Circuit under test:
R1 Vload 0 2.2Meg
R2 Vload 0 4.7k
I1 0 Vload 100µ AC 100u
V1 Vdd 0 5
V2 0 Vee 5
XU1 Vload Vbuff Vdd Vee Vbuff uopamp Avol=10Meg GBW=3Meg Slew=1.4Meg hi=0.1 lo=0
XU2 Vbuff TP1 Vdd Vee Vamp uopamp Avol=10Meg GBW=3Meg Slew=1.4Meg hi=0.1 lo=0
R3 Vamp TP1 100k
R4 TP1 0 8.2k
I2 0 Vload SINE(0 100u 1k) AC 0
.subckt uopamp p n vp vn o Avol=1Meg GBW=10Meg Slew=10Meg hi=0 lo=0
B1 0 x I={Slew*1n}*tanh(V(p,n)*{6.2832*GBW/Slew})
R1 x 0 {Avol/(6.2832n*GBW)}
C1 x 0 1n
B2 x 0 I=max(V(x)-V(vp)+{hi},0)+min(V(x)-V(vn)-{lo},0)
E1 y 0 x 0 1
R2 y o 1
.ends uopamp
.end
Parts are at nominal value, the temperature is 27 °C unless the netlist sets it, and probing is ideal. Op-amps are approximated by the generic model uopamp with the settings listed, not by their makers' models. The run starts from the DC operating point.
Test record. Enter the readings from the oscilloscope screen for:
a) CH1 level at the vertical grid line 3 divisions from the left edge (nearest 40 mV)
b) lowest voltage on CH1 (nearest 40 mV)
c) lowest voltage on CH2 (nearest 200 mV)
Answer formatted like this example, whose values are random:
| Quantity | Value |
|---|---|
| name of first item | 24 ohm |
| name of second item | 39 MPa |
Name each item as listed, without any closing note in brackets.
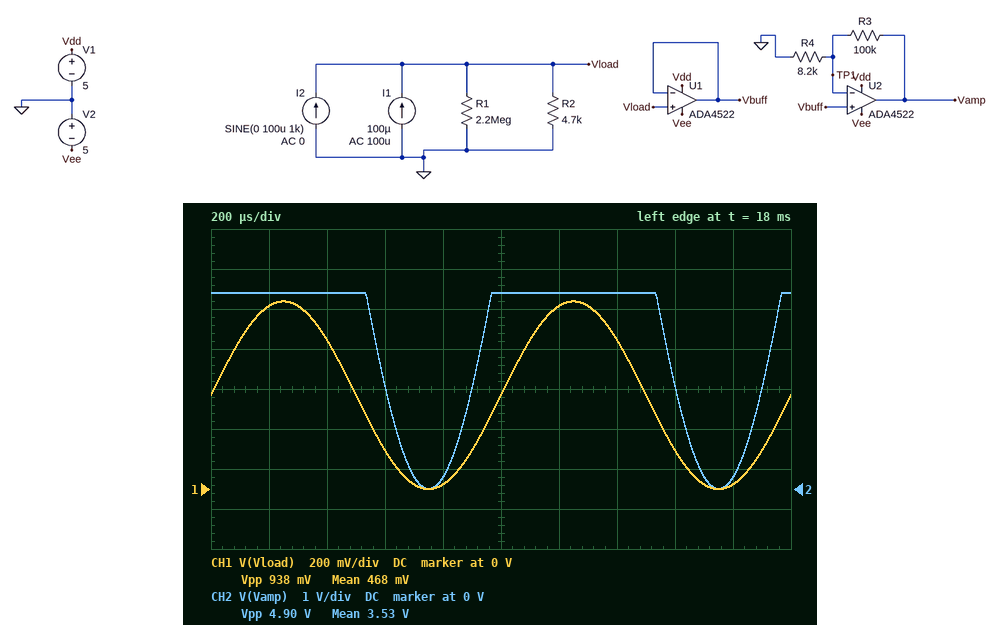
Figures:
| Quantity | Value |
|---|---|
| CH1 level at the vertical grid line 3 divisions from the left edge | 200 mV |
| lowest voltage on CH1 | 0 V |
| lowest voltage on CH2 | 0 V |
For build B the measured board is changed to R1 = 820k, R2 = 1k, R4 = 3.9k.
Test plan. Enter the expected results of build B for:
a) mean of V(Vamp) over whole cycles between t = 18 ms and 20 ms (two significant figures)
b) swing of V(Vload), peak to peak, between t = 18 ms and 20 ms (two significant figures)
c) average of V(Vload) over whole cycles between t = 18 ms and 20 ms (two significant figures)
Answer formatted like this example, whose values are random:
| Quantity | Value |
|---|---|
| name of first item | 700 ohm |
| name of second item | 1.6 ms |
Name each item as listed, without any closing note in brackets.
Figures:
| Quantity | Value |
|---|---|
| mean of V(Vamp) over whole cycles between t = 18 ms and 20 ms | 2.6 V |
| swing of V(Vload), peak to peak, between t = 18 ms and 20 ms | 200 mV |
| average of V(Vload) over whole cycles between t = 18 ms and 20 ms | 100 mV |
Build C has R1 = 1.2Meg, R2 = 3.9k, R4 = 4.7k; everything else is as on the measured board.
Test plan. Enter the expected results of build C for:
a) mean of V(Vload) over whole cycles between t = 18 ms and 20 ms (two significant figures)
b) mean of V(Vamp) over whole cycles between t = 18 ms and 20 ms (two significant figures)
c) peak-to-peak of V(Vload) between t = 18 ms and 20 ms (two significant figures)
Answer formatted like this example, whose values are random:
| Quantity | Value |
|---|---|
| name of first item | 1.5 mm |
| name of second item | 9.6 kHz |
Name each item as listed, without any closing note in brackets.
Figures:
| Quantity | Value |
|---|---|
| mean of V(Vload) over whole cycles between t = 18 ms and 20 ms | 390 mV |
| mean of V(Vamp) over whole cycles between t = 18 ms and 20 ms | 3.8 V |
| peak-to-peak of V(Vload) between t = 18 ms and 20 ms | 780 mV |
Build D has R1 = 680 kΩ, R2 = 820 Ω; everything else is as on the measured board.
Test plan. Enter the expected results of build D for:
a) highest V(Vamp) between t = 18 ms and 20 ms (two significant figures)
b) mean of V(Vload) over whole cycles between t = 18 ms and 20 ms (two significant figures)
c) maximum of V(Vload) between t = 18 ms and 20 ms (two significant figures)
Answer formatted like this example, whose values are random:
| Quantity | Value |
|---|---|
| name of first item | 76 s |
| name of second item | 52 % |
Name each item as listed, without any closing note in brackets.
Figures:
| Quantity | Value |
|---|---|
| highest V(Vamp) between t = 18 ms and 20 ms | 2.2 V |
| mean of V(Vload) over whole cycles between t = 18 ms and 20 ms | 82 mV |
| maximum of V(Vload) between t = 18 ms and 20 ms | 160 mV |
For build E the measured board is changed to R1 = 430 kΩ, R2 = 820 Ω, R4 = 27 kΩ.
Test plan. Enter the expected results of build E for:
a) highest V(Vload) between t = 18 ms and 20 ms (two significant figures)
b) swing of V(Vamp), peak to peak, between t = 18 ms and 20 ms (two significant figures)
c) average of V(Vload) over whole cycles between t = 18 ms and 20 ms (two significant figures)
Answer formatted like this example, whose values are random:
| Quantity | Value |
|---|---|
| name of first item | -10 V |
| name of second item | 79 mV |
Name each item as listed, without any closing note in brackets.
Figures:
| Quantity | Value |
|---|---|
| highest V(Vload) between t = 18 ms and 20 ms | 160 mV |
| swing of V(Vamp), peak to peak, between t = 18 ms and 20 ms | 770 mV |
| average of V(Vload) over whole cycles between t = 18 ms and 20 ms | 82 mV |
